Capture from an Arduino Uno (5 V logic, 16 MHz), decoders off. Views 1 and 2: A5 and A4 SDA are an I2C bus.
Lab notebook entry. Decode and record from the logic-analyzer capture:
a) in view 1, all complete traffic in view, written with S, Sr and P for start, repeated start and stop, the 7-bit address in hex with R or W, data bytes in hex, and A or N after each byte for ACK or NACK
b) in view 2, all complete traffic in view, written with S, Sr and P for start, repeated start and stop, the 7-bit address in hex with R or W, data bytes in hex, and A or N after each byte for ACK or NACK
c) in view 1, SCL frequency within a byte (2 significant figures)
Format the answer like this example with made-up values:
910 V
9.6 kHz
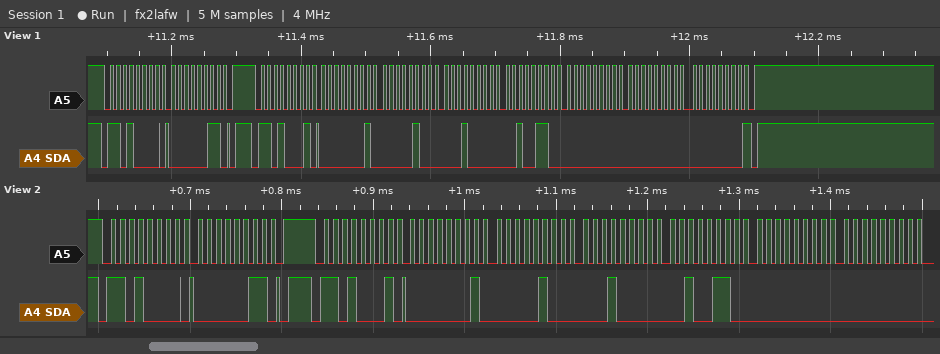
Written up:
S 68W A 03 A P S 68R A 01 A 04 A 10 A 26 A 00 A 00 A 00 N P
S 68W A 03 A P S 68R A 01 A 04 A 10 A 26 A 00 A 00 A
100 kHz
